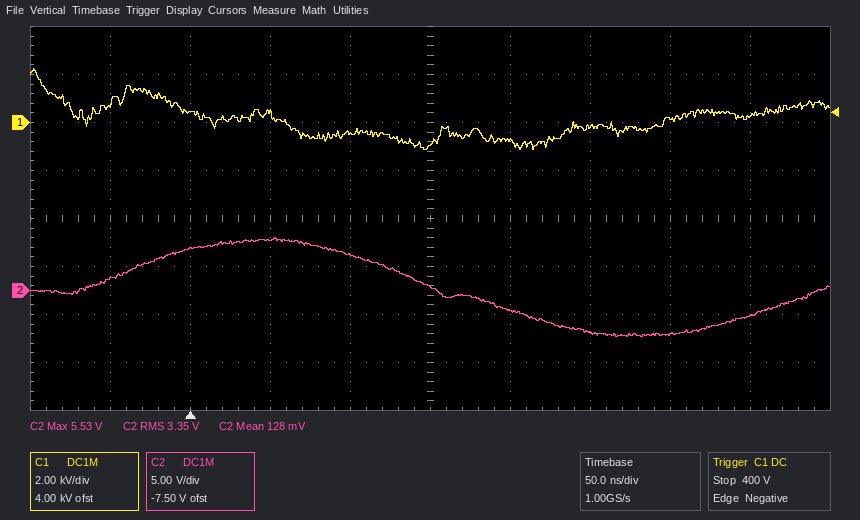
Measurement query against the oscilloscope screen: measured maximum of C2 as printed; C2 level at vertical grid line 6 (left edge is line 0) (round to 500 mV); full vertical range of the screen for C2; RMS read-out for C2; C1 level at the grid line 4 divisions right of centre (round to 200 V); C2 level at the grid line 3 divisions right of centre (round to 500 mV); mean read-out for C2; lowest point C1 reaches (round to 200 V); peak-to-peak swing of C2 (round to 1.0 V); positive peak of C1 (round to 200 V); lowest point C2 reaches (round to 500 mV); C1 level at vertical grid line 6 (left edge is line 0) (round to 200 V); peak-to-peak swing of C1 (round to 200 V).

5.53 V
-2.0 V
40 V
3.35 V
200 V
-4.5 V
128 mV
-1.2 kV
10.0 V
2.2 kV
-5.0 V
-800 V
3.4 kV
